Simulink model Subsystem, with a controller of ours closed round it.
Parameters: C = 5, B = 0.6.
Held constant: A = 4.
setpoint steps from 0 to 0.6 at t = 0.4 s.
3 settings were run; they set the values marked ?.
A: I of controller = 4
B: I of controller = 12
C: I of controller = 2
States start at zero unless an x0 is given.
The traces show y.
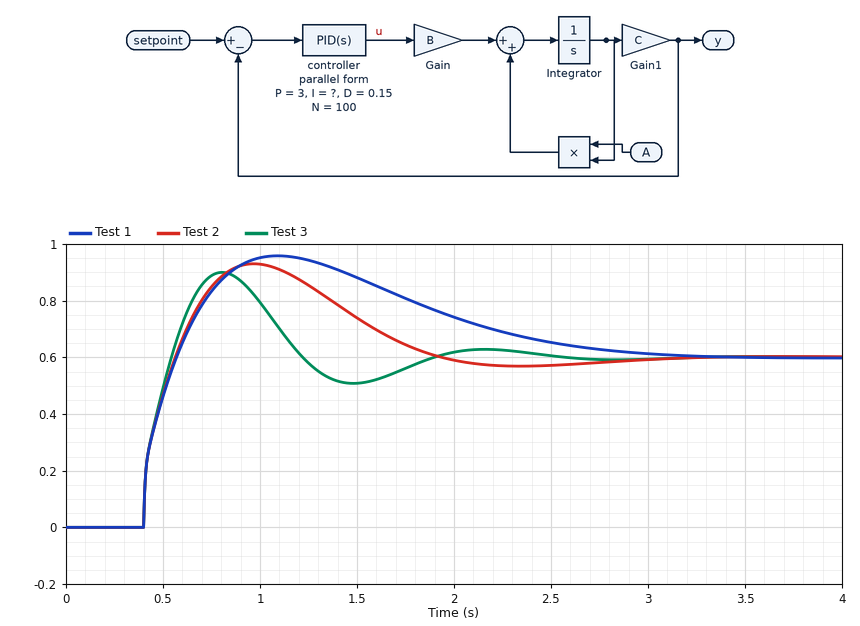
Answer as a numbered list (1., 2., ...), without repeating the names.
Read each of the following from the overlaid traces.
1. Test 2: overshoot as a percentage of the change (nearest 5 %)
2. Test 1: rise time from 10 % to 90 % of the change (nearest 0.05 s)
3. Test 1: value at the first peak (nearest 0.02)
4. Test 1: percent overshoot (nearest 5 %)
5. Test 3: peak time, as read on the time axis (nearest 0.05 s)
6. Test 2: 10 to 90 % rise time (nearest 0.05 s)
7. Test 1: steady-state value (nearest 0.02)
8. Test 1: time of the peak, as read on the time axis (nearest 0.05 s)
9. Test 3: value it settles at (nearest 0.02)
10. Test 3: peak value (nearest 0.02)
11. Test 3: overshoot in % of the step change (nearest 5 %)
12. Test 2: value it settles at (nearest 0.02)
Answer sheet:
1. 55 %
2. 0.15 s
3. 0.96
4. 60 %
5. 0.80 s
6. 0.15 s
7. 0.60
8. 1.10 s
9. 0.60
10. 0.90
11. 50 %
12. 0.60
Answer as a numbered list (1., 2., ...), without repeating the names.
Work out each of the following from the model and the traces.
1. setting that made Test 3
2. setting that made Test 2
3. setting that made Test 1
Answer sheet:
1. B
2. A
3. C
